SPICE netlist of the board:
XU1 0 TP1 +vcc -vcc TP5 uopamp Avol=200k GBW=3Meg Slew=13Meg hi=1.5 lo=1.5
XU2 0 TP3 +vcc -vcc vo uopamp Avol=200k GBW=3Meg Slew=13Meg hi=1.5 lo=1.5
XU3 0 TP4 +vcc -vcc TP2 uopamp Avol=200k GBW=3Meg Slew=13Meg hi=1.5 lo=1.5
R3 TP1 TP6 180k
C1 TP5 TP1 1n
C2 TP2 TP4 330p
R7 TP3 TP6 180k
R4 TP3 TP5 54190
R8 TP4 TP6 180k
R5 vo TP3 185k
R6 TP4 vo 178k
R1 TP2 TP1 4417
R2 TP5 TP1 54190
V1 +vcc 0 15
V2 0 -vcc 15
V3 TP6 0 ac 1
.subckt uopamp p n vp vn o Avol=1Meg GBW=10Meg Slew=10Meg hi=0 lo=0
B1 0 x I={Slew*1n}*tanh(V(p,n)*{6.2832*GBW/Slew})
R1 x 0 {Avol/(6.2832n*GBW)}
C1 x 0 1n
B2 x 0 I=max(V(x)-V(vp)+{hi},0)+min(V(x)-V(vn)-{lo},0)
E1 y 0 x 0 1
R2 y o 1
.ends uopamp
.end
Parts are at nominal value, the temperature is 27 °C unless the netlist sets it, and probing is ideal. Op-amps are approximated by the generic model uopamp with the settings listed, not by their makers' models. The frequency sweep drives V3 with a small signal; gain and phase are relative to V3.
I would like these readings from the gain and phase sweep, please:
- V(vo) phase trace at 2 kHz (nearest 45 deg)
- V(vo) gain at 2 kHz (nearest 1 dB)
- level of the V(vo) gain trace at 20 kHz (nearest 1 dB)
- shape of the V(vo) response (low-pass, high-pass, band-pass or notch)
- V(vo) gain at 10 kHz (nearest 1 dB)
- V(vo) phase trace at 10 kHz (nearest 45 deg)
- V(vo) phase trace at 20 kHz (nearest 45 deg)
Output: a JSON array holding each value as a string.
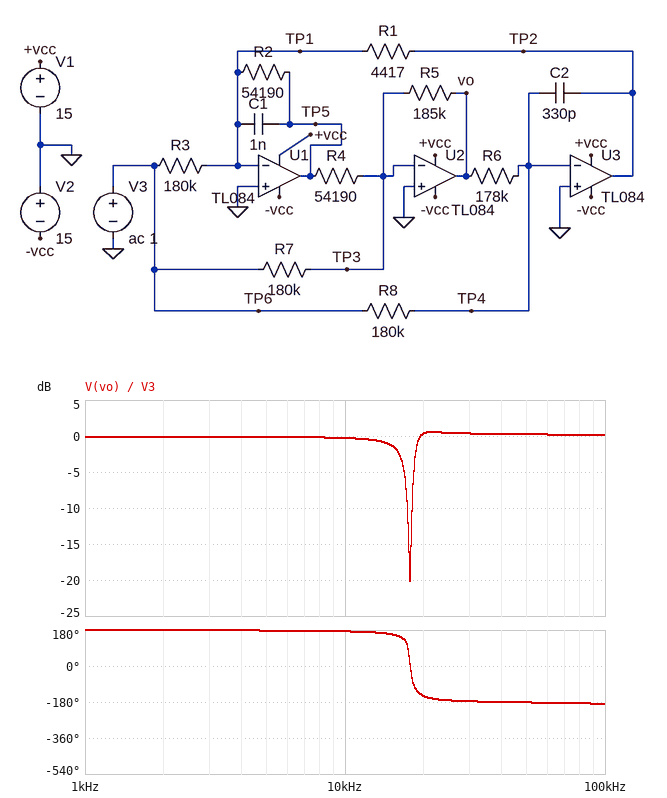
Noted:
["180 deg", "0 dB", "0 dB", "notch", "0 dB", "180 deg", "-135 deg"]
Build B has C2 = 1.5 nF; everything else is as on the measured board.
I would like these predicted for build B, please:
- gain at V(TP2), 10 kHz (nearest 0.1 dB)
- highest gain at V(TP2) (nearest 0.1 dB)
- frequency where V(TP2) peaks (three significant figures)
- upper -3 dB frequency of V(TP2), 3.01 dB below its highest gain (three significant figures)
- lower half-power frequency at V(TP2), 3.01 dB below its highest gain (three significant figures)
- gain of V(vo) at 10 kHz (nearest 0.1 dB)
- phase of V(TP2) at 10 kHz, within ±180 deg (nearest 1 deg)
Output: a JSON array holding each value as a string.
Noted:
["-27.6 dB", "-22.9 dB", "8.27 kHz", "9.54 kHz", "6.72 kHz", "-1.9 dB", "36 deg"]
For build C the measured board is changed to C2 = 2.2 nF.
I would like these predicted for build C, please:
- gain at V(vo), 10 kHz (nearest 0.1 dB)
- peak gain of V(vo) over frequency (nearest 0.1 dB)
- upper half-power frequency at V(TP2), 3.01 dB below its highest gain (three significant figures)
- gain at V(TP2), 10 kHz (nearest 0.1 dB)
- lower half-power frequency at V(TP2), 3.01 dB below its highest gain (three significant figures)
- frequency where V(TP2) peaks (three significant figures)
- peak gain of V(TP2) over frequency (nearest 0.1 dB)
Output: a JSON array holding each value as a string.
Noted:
["-0.6 dB", "0.2 dB", "8.01 kHz", "-34.4 dB", "5.09 kHz", "6.73 kHz", "-24.5 dB"]
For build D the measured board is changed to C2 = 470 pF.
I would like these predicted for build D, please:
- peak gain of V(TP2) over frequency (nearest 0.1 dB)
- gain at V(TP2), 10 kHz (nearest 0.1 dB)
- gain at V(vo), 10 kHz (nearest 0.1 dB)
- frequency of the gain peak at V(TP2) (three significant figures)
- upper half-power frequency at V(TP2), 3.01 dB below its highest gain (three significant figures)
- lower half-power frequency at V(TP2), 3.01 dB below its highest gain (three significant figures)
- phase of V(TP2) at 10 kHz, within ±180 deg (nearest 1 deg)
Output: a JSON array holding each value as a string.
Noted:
["-17.4 dB", "-28.2 dB", "-0.5 dB", "15.1 kHz", "16.2 kHz", "13.8 kHz", "161 deg"]
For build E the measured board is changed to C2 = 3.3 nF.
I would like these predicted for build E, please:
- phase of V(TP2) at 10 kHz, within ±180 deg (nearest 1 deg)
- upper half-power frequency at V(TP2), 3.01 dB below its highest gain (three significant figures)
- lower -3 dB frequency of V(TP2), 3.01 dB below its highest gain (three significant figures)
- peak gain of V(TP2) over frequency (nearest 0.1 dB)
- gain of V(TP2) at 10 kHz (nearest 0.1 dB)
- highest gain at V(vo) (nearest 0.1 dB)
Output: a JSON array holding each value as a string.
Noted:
["14 deg", "6.66 kHz", "3.60 kHz", "-26.2 dB", "-39.9 dB", "0.2 dB"]
